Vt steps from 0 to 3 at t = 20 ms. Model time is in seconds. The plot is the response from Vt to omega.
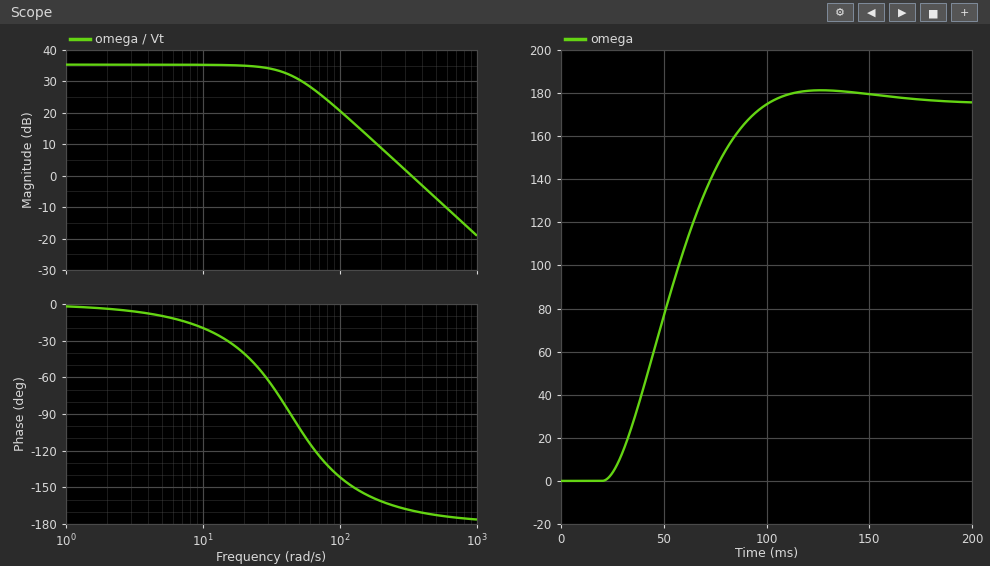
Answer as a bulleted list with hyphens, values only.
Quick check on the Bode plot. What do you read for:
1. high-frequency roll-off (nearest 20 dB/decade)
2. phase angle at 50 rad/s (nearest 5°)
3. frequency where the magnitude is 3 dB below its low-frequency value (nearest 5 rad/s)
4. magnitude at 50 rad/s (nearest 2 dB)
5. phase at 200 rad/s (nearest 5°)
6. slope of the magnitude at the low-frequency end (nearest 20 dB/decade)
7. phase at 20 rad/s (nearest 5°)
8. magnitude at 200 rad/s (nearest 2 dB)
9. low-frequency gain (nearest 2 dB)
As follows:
- -40 dB/decade
- -100°
- 40 rad/s
- 30 dB
- -160°
- 0 dB/decade
- -40°
- 8 dB
- 36 dB
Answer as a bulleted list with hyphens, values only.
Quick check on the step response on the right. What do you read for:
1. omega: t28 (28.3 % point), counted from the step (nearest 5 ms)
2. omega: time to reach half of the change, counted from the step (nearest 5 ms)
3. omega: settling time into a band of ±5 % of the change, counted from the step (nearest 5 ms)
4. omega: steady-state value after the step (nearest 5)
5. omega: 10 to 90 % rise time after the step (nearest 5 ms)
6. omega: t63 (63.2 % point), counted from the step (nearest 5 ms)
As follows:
- 20 ms
- 35 ms
- 70 ms
- 175
- 50 ms
- 40 ms
